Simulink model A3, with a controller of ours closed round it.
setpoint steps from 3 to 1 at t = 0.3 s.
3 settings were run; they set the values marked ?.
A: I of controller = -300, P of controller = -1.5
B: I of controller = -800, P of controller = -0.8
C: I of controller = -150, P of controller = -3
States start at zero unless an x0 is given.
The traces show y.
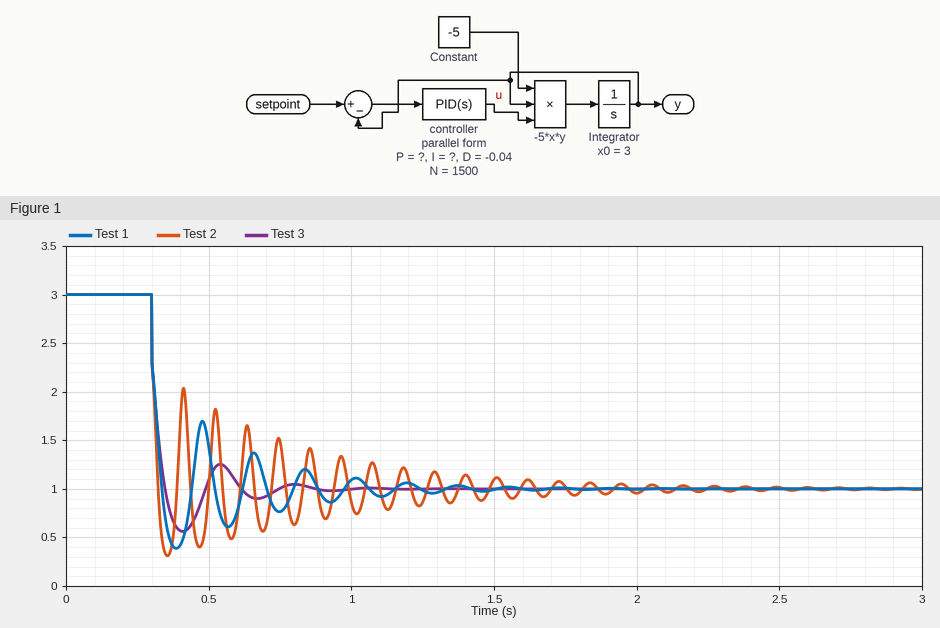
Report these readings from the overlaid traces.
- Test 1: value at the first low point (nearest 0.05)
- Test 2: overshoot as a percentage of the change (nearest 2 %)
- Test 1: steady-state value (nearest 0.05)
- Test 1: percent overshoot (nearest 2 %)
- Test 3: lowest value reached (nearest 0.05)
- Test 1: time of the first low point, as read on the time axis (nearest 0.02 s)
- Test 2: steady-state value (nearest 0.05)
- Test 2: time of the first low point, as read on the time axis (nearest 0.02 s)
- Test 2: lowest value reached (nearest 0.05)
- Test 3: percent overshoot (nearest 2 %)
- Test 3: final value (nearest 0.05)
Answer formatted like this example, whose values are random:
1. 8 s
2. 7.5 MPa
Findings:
1. 0.40
2. 34 %
3. 1.00
4. 30 %
5. 0.55
6. 0.38 s
7. 1.00
8. 0.36 s
9. 0.30
10. 22 %
11. 1.00
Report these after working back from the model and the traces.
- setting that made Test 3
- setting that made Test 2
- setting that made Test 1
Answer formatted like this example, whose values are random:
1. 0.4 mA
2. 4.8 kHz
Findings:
1. C
2. B
3. A
